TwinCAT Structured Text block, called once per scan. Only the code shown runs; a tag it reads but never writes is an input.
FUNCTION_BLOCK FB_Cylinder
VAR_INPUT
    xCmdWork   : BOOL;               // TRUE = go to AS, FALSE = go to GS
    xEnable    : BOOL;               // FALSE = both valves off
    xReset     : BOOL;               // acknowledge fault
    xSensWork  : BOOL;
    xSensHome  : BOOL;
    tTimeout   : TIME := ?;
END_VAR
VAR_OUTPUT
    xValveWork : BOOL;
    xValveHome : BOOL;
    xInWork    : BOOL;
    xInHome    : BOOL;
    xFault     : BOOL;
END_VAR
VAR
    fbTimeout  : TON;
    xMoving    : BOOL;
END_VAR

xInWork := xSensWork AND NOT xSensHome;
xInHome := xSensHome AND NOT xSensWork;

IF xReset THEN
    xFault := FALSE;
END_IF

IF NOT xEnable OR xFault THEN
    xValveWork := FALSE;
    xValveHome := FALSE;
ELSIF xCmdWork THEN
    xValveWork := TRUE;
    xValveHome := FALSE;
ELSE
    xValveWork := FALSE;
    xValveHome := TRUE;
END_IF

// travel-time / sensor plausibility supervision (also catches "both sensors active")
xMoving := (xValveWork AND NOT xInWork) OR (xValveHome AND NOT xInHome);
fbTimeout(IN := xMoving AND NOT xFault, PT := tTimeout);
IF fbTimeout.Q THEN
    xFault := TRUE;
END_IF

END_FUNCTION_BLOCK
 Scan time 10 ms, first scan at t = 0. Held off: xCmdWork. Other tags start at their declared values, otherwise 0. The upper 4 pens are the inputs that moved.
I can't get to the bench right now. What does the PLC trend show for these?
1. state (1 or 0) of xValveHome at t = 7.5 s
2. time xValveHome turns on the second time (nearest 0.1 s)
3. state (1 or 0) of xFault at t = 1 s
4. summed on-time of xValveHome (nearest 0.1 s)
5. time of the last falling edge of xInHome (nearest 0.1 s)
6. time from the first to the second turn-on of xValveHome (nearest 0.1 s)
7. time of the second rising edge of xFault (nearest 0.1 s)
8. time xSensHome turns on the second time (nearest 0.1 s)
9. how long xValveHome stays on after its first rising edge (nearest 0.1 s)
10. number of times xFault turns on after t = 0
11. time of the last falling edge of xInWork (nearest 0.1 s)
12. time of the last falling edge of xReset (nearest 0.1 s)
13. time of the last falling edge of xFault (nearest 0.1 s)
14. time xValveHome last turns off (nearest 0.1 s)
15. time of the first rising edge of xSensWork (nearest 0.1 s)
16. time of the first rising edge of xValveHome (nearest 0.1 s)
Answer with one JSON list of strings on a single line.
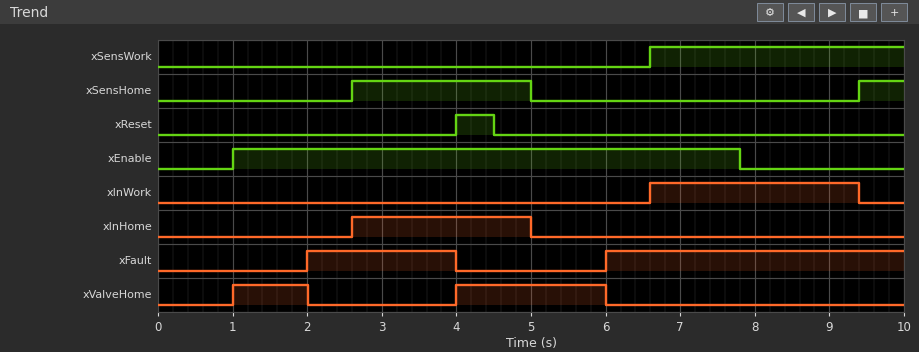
["0", "4.0 s", "0", "3.0 s", "5.0 s", "3.0 s", "6.0 s", "9.4 s", "1.0 s", "2", "9.4 s", "4.5 s", "4.0 s", "6.0 s", "6.6 s", "1.0 s"]
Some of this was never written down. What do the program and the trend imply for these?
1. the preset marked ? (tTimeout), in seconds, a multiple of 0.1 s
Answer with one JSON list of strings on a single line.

["1.0 s"]
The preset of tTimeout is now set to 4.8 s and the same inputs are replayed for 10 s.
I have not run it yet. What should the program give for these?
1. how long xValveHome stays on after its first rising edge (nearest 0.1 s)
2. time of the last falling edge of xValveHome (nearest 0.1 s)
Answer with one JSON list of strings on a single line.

["6.8 s", "7.8 s"]
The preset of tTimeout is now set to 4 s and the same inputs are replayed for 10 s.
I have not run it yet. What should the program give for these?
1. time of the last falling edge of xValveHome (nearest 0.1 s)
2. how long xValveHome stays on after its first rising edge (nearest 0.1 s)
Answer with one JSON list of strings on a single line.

["7.8 s", "6.8 s"]
